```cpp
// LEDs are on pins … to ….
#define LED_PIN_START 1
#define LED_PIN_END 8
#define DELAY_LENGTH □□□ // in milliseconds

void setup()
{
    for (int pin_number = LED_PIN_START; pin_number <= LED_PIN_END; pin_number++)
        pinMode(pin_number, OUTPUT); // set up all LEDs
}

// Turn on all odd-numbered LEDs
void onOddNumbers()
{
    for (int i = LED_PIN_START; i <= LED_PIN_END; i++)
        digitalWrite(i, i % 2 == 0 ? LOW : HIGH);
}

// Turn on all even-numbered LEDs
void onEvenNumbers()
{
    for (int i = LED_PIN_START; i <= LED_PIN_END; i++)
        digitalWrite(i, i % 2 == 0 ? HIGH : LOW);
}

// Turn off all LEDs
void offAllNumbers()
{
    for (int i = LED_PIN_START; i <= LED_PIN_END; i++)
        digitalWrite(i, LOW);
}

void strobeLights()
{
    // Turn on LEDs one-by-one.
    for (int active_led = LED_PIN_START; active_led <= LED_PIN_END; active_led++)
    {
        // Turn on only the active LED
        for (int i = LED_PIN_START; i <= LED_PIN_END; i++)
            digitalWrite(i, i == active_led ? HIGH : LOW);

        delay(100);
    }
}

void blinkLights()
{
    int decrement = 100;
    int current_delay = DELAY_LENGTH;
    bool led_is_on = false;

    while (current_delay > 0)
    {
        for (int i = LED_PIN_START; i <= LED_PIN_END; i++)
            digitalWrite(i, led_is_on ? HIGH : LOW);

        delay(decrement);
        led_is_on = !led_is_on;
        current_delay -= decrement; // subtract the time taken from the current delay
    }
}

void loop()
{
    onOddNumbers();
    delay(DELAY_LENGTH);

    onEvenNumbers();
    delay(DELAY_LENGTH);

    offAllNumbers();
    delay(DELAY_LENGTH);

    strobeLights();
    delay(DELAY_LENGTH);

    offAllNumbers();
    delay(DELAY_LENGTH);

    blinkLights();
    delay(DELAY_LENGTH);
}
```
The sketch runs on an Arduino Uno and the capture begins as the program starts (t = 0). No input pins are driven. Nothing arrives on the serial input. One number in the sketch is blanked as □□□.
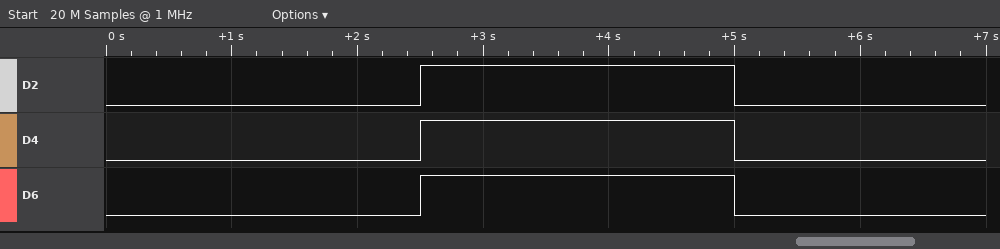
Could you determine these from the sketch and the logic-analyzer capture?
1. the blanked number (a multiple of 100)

2500
